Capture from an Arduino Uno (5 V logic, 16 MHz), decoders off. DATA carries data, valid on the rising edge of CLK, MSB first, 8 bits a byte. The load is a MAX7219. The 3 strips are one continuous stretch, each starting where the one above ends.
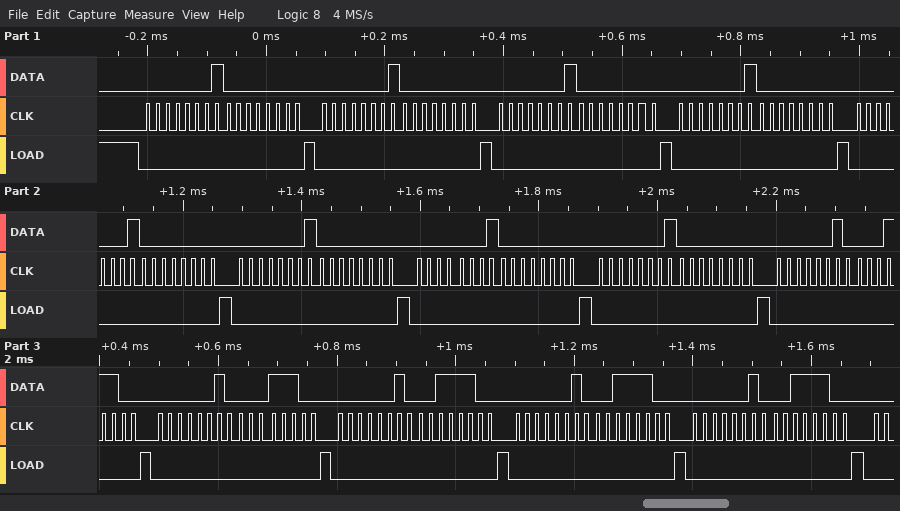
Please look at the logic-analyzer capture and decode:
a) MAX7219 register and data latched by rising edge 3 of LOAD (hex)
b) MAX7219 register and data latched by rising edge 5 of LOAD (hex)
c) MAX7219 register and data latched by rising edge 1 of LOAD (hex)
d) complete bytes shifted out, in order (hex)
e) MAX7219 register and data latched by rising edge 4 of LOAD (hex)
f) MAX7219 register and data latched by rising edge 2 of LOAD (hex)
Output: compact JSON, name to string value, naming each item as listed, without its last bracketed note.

{"MAX7219 register and data latched by rising edge 3 of LOAD": "register 0x1, data 0x00", "MAX7219 register and data latched by rising edge 5 of LOAD": "register 0x1, data 0x00", "MAX7219 register and data latched by rising edge 1 of LOAD": "register 0x1, data 0x00", "complete bytes shifted out, in order": "01 00 01 00 01 00 01 00 01 00 01 00 01 00 01 00 02 1C 02 1C 02 3C 02 3C 02 3C", "MAX7219 register and data latched by rising edge 4 of LOAD": "register 0x1, data 0x00", "MAX7219 register and data latched by rising edge 2 of LOAD": "register 0x1, data 0x00"}
